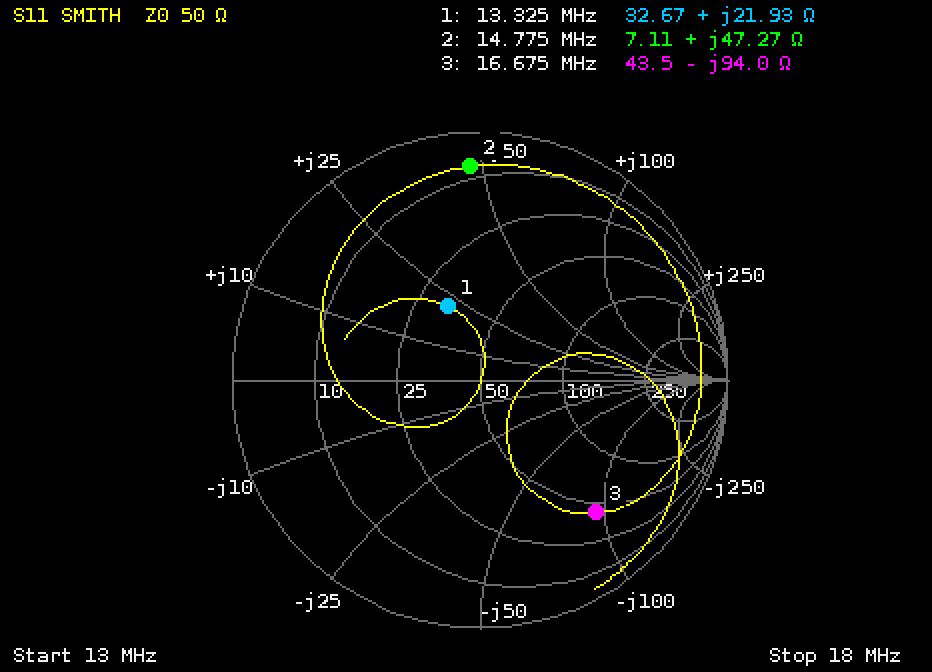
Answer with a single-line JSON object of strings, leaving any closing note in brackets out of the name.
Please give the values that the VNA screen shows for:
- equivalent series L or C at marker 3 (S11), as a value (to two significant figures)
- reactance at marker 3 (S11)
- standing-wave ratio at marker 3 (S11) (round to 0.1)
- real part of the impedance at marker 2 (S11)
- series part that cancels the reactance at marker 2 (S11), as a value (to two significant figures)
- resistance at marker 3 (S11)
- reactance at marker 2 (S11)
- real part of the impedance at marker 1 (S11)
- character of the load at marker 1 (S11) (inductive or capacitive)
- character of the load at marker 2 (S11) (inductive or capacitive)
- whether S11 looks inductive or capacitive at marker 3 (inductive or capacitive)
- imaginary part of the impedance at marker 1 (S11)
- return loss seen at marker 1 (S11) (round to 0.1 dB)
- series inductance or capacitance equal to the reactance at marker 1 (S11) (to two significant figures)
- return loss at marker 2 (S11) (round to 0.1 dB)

{"equivalent series L or C at marker 3 (S11), as a value": "100 pF", "reactance at marker 3": "-94.0 Ω", "standing-wave ratio at marker 3 (S11)": "5.9", "real part of the impedance at marker 2": "7.11 Ω", "series part that cancels the reactance at marker 2 (S11), as a value": "230 pF", "resistance at marker 3": "43.5 Ω", "reactance at marker 2": "+47.27 Ω", "real part of the impedance at marker 1": "32.67 Ω", "character of the load at marker 1 (S11)": "inductive", "character of the load at marker 2 (S11)": "inductive", "whether S11 looks inductive or capacitive at marker 3": "capacitive", "imaginary part of the impedance at marker 1": "+21.93 Ω", "return loss seen at marker 1 (S11)": "9.7 dB", "series inductance or capacitance equal to the reactance at marker 1 (S11)": "260 nH", "return loss at marker 2 (S11)": "1.3 dB"}
